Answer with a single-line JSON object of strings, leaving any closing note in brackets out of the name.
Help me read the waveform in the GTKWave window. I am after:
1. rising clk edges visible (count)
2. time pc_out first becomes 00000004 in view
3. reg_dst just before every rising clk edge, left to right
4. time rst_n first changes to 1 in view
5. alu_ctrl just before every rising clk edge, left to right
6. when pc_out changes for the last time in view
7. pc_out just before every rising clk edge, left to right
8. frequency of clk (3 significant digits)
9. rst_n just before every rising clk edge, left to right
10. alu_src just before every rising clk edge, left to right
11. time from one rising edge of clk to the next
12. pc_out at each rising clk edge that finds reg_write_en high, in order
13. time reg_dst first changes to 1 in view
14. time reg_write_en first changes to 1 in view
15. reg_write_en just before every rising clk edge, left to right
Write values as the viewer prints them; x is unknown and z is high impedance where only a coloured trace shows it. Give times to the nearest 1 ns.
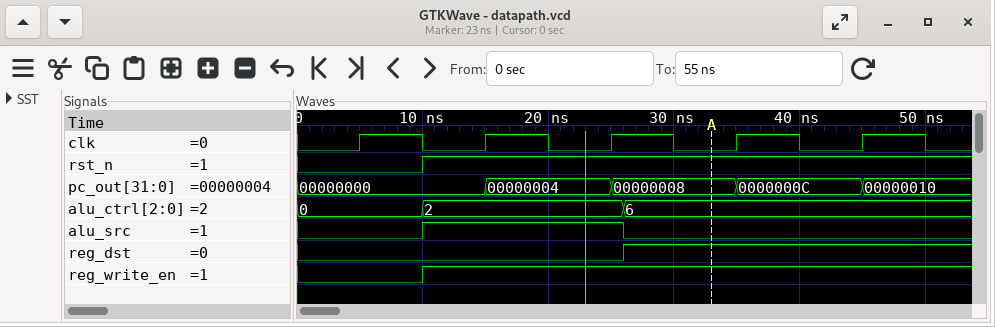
{"rising clk edges visible": "5", "time pc_out first becomes 00000004 in view": "15 ns", "reg_dst just before every rising clk edge, left to right": "0 0 0 1 1", "time rst_n first changes to 1 in view": "10 ns", "alu_ctrl just before every rising clk edge, left to right": "0, 2, 2, 6, 6", "when pc_out changes for the last time in view": "45 ns", "pc_out just before every rising clk edge, left to right": "00000000, 00000000, 00000004, 00000008, 0000000C", "frequency of clk": "100 MHz", "rst_n just before every rising clk edge, left to right": "0 1 1 1 1", "alu_src just before every rising clk edge, left to right": "0 1 1 0 0", "time from one rising edge of clk to the next": "10 ns", "pc_out at each rising clk edge that finds reg_write_en high, in order": "00000000, 00000004, 00000008, 0000000C", "time reg_dst first changes to 1 in view": "26 ns", "time reg_write_en first changes to 1 in view": "10 ns", "reg_write_en just before every rising clk edge, left to right": "0 1 1 1 1"}
